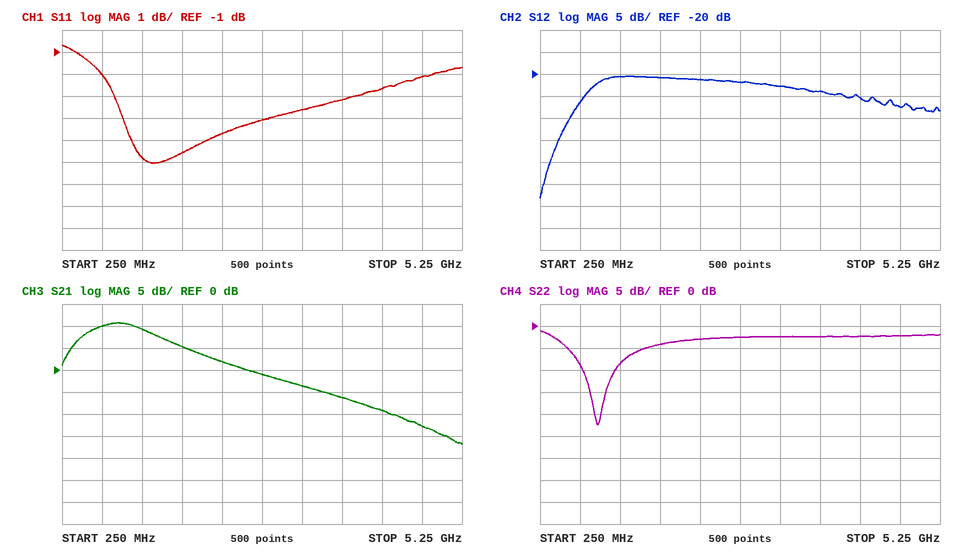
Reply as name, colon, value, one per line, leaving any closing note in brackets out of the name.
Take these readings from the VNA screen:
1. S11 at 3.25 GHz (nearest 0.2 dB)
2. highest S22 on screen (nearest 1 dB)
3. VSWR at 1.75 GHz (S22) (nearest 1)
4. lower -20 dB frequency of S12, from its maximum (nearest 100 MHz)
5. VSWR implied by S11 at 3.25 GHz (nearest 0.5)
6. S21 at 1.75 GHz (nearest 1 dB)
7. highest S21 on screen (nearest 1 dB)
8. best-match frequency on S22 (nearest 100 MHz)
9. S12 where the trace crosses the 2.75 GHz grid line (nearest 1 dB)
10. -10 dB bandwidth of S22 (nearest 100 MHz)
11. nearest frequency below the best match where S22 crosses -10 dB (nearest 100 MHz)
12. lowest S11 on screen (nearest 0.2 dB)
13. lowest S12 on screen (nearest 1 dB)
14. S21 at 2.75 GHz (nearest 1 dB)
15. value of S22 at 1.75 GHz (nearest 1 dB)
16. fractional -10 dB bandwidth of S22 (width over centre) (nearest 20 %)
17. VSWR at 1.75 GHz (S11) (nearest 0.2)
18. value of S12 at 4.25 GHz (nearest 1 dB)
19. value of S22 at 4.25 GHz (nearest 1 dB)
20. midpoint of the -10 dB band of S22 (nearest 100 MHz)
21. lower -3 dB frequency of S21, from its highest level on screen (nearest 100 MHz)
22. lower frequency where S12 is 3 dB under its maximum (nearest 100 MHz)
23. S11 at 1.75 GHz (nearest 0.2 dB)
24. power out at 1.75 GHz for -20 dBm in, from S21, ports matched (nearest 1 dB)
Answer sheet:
S11 at 3.25 GHz: -3.6 dB
highest S22 on screen: -1 dB
VSWR at 1.75 GHz (S22): 4
lower -20 dB frequency of S12, from its maximum: 400 MHz
VSWR implied by S11 at 3.25 GHz: 5.0
S21 at 1.75 GHz: 5 dB
highest S21 on screen: 11 dB
best-match frequency on S22: 1.0 GHz
S12 where the trace crosses the 2.75 GHz grid line: -22 dB
-10 dB bandwidth of S22: 400 MHz
nearest frequency below the best match where S22 crosses -10 dB: 800 MHz
lowest S11 on screen: -6.0 dB
lowest S12 on screen: -48 dB
S21 at 2.75 GHz: -1 dB
value of S22 at 1.75 GHz: -4 dB
fractional -10 dB bandwidth of S22 (width over centre): 40 %
VSWR at 1.75 GHz (S11): 3.2
value of S12 at 4.25 GHz: -25 dB
value of S22 at 4.25 GHz: -2 dB
midpoint of the -10 dB band of S22: 1.0 GHz
lower -3 dB frequency of S21, from its highest level on screen: 500 MHz
lower frequency where S12 is 3 dB under its maximum: 900 MHz
S11 at 1.75 GHz: -5.6 dB
power out at 1.75 GHz for -20 dBm in, from S21, ports matched: -15 dBm
